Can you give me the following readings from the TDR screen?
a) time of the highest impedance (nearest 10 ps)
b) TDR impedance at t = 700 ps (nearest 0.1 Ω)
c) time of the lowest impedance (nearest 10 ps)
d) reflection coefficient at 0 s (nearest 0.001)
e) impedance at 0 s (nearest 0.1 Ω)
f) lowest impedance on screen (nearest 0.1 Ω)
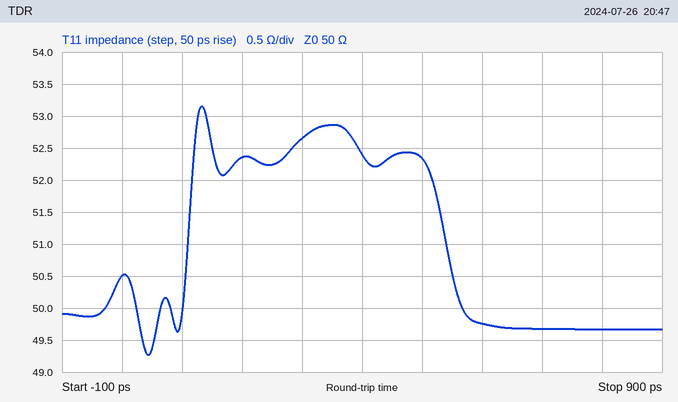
130 ps
49.7 Ω
40 ps
+0.005
50.5 Ω
49.3 Ω
